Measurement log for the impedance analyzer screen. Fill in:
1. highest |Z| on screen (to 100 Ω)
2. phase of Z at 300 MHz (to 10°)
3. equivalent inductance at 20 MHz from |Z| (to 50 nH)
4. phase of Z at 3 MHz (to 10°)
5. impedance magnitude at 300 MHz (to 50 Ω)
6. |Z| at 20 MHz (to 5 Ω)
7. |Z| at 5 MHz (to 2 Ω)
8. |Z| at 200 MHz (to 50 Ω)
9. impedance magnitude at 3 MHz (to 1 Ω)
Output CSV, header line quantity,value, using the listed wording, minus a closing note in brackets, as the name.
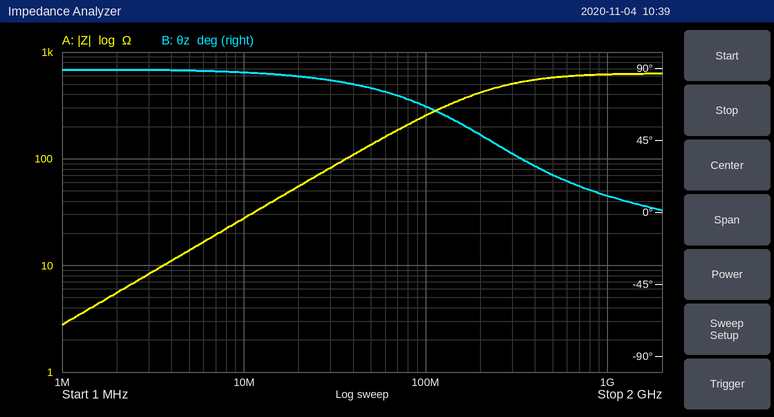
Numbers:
quantity,value
highest |Z| on screen,600 Ω
phase of Z at 300 MHz,40°
equivalent inductance at 20 MHz from |Z|,450 nH
phase of Z at 3 MHz,90°
impedance magnitude at 300 MHz,500 Ω
|Z| at 20 MHz,55 Ω
|Z| at 5 MHz,14 Ω
|Z| at 200 MHz,400 Ω
impedance magnitude at 3 MHz,8 Ω
